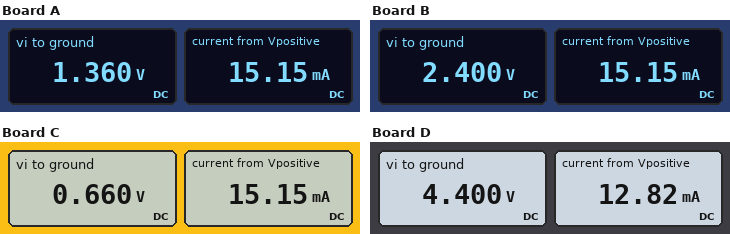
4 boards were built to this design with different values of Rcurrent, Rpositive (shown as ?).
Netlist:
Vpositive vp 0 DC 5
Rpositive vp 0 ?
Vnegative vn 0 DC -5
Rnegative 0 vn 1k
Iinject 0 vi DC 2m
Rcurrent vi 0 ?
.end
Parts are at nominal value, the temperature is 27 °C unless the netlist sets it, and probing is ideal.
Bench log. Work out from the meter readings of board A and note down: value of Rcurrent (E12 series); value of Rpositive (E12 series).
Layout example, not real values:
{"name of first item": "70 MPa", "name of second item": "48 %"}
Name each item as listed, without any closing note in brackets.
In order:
{"value of Rcurrent": "680 Ω", "value of Rpositive": "330 Ω"}
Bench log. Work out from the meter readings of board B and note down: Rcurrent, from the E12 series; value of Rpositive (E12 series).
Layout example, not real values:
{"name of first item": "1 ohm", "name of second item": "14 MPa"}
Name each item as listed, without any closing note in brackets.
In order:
{"Rcurrent, from the E12 series": "1.2 kΩ", "value of Rpositive": "330 Ω"}
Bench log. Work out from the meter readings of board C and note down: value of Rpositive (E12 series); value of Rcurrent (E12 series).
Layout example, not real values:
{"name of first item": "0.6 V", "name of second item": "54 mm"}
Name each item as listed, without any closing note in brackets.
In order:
{"value of Rpositive": "330 Ω", "value of Rcurrent": "330 Ω"}
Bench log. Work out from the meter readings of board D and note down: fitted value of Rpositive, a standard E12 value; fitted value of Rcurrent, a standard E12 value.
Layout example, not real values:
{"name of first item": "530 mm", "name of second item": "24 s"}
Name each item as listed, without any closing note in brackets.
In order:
{"fitted value of Rpositive, a standard E12 value": "390 Ω", "fitted value of Rcurrent, a standard E12 value": "2.2 kΩ"}
